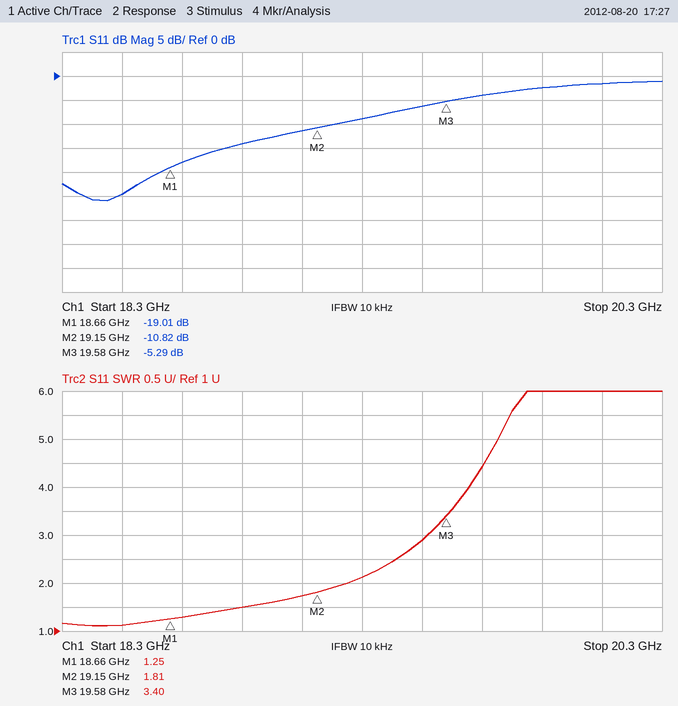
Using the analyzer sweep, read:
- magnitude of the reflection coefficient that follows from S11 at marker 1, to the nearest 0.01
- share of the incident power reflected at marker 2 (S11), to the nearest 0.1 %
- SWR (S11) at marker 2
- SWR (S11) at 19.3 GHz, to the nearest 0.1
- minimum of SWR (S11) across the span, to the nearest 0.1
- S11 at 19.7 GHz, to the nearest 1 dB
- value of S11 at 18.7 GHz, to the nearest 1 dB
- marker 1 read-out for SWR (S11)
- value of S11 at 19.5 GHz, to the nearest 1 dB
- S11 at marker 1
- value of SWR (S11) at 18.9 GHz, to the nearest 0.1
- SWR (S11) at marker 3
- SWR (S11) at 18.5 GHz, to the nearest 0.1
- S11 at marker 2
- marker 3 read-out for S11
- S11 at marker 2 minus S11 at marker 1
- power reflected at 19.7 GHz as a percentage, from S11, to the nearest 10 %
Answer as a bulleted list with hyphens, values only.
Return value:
- 0.11
- 8.3 %
- 1.81
- 2.1
- 1.1
- -4 dB
- -18 dB
- 1.25
- -6 dB
- -19.01 dB
- 1.5
- 3.40
- 1.1
- -10.82 dB
- -5.29 dB
- 8.19 dB
- 40 %
